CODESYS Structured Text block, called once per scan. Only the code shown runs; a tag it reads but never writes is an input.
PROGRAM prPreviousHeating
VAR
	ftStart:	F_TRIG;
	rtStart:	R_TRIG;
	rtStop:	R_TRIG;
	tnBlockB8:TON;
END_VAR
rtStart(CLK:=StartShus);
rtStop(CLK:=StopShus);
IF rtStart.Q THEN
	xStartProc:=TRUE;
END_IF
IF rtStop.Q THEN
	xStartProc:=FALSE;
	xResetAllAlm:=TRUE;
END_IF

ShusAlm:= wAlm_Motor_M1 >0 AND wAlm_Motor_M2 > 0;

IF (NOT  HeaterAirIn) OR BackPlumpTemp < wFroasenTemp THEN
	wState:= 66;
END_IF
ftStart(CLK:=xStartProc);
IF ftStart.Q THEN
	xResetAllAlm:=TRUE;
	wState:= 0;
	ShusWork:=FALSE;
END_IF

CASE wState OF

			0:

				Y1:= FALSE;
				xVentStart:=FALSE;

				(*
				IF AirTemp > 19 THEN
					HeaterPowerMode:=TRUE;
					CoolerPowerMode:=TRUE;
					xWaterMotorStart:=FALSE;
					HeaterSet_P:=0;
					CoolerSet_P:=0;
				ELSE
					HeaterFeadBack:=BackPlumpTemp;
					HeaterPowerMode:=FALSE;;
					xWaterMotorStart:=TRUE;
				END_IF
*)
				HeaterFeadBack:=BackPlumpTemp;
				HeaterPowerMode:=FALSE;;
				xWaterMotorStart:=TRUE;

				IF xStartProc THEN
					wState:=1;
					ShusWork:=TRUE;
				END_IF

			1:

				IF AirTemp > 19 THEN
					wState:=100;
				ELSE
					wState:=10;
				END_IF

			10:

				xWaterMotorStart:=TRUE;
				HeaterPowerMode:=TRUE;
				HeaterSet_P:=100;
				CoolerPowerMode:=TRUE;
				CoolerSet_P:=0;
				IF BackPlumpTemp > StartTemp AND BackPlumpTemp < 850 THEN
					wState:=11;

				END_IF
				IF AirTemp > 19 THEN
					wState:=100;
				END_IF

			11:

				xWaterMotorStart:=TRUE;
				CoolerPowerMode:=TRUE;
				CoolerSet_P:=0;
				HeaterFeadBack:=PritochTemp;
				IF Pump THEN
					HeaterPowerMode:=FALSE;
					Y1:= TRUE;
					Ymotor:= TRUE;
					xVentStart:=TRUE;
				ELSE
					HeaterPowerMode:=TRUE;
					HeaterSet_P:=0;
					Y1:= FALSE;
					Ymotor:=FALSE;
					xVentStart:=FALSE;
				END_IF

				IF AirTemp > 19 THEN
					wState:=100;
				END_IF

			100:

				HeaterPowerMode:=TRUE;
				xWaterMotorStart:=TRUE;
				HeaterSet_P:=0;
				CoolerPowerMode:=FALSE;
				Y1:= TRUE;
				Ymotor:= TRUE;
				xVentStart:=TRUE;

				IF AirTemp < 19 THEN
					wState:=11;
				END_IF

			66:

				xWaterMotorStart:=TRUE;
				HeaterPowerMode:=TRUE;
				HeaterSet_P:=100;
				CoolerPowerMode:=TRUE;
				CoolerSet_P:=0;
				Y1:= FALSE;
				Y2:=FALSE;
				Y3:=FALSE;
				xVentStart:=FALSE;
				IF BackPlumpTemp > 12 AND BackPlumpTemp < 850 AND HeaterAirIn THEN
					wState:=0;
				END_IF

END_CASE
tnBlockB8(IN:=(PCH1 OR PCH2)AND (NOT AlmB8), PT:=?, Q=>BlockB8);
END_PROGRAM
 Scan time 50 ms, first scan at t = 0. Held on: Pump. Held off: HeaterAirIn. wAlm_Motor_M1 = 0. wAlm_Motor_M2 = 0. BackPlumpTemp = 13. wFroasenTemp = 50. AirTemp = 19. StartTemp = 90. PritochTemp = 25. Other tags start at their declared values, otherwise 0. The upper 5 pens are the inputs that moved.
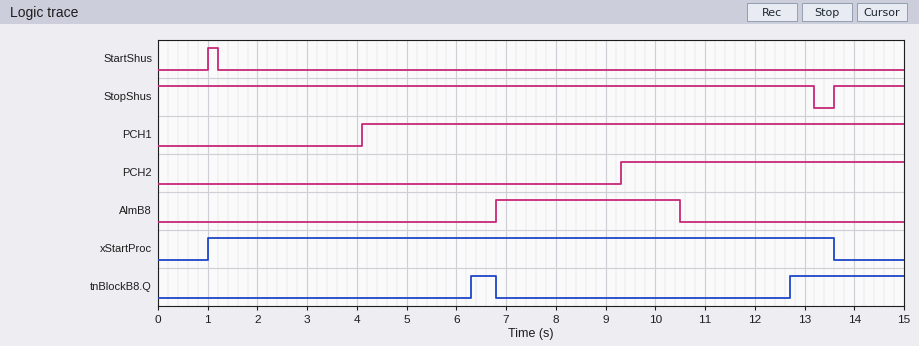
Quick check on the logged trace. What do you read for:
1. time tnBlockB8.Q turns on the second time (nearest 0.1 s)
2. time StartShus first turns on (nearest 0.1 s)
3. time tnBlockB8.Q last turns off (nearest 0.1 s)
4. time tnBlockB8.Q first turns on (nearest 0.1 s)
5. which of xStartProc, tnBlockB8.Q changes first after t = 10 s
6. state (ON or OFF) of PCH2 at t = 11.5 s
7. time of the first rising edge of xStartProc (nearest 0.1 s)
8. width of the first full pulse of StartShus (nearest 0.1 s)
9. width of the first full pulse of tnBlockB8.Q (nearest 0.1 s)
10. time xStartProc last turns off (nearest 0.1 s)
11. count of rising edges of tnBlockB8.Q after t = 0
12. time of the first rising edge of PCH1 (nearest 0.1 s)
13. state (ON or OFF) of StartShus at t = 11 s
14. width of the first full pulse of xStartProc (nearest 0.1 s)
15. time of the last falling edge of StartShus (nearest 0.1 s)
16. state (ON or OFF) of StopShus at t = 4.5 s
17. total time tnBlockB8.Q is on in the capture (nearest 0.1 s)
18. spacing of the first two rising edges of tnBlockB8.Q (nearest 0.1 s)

12.7 s
1.0 s
6.8 s
6.3 s
tnBlockB8.Q
ON
1.0 s
0.2 s
0.5 s
13.6 s
2
4.1 s
OFF
12.6 s
1.2 s
ON
2.8 s
6.4 s
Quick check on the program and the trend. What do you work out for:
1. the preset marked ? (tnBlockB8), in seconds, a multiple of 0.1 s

2.2 s
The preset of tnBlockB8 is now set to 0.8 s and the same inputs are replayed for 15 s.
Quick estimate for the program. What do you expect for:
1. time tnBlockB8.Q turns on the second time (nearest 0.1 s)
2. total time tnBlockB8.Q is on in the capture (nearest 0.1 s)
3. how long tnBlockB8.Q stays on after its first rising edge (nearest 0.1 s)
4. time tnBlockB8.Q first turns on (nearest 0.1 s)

11.3 s
5.6 s
1.9 s
4.9 s
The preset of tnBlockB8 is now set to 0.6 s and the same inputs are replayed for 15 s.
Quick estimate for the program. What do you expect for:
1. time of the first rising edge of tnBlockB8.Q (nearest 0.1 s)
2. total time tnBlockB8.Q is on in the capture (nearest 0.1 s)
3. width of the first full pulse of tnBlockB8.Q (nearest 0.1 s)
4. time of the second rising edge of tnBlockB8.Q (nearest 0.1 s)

4.7 s
6.0 s
2.1 s
11.1 s
